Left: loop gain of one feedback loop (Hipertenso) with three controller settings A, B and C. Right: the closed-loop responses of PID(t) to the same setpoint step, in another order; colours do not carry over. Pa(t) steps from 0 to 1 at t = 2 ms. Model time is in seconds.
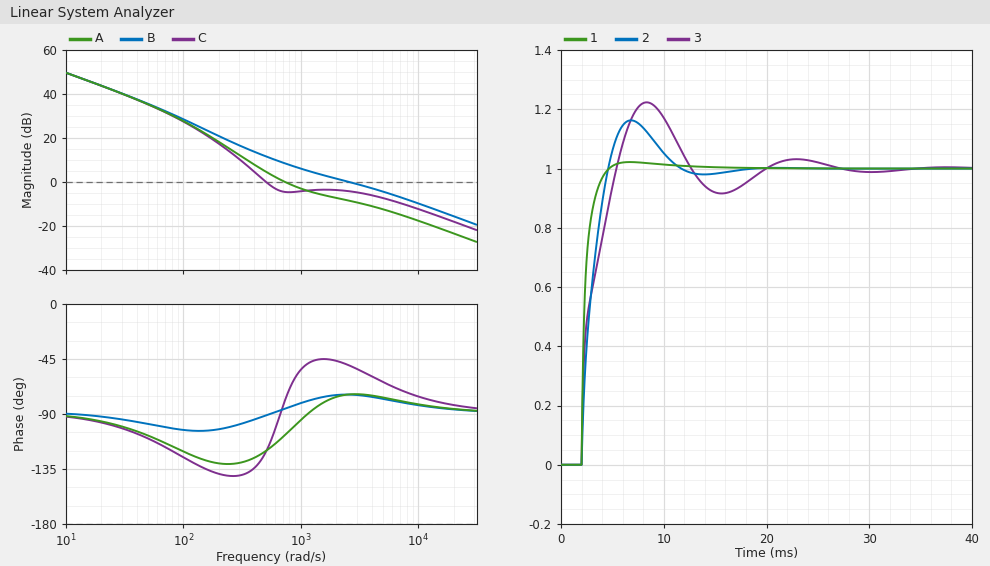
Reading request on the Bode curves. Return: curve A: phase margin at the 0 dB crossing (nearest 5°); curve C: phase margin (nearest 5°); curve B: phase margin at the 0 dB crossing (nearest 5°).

75°
60°
105°
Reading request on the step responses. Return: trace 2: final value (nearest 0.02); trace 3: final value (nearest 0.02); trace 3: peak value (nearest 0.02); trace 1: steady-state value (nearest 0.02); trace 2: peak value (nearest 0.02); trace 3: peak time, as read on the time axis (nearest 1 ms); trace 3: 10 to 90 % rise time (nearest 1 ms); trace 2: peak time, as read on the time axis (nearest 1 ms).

1.00
1.00
1.22
1.00
1.16
8 ms
3 ms
7 ms
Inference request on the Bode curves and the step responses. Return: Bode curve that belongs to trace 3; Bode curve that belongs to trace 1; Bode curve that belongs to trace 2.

C
B
A
